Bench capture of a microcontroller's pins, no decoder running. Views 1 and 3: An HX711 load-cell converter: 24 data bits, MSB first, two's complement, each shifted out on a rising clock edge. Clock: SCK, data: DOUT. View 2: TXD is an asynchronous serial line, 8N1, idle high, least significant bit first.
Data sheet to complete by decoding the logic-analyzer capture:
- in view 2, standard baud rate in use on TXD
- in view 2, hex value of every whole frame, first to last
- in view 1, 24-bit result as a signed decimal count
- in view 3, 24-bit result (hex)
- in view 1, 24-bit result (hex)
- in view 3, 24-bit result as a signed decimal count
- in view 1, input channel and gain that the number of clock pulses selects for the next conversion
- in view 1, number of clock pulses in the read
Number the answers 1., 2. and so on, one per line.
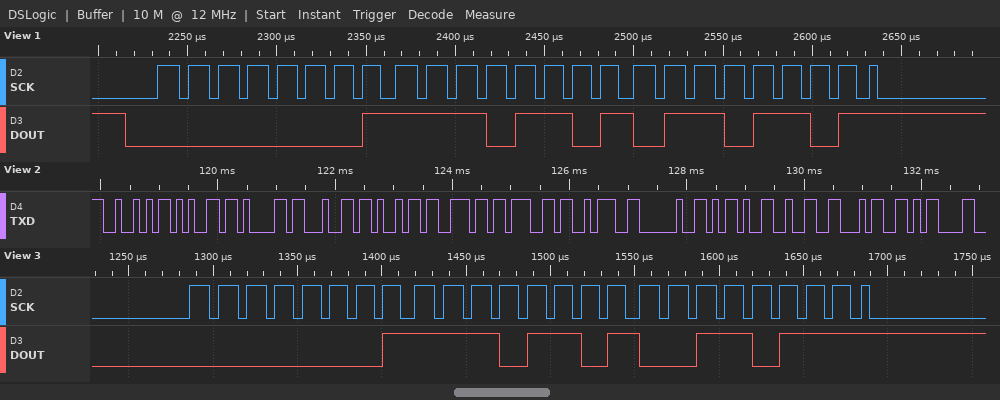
1. 9600 baud
2. 52 65 61 64 69 6E 67 3A 20 2D 32 34 0D
3. 126317
4. 0x01ED37
5. 0x01ED6D
6. 126263
7. channel A, gain 128
8. 25
